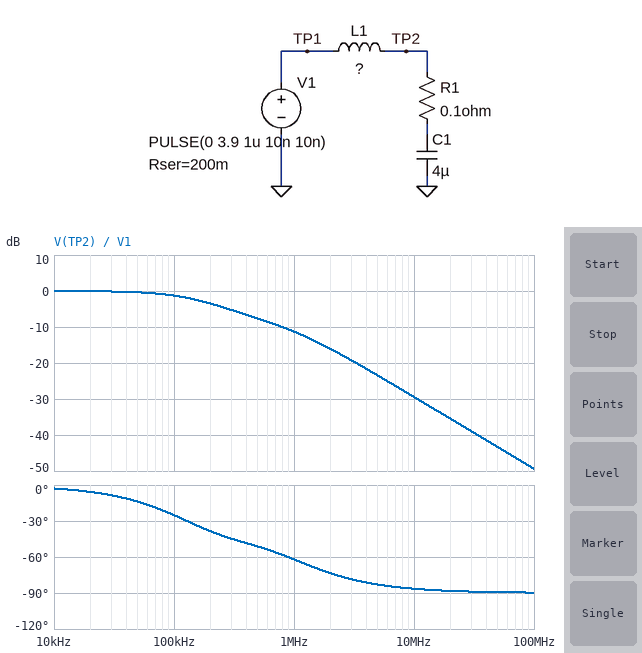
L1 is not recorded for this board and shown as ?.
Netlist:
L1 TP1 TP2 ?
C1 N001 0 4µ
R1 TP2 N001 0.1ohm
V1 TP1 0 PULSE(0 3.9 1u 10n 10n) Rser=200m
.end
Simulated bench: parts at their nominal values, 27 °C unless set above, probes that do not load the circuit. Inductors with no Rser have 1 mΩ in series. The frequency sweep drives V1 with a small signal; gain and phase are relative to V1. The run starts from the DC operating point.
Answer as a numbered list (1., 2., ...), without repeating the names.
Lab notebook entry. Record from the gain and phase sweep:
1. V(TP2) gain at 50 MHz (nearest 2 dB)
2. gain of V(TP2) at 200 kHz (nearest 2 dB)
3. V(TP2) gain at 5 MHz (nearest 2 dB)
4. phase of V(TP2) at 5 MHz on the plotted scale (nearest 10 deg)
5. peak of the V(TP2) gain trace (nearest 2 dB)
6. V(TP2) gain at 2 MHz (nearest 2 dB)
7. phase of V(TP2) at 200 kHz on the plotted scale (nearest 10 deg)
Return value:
1. -44 dB
2. -4 dB
3. -24 dB
4. -80 deg
5. 0 dB
6. -16 dB
7. -40 deg
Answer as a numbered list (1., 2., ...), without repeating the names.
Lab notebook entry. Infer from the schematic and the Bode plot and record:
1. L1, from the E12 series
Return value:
1. 47 nH
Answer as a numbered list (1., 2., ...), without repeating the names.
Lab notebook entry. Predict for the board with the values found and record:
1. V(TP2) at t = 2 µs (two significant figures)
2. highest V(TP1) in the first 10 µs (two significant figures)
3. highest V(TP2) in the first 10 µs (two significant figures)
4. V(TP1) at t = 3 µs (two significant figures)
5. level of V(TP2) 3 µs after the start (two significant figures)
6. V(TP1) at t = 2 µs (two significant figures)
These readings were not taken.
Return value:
1. 2.8 V
2. 3.9 V
3. 3.9 V
4. 3.4 V
5. 3.5 V
6. 2.5 V
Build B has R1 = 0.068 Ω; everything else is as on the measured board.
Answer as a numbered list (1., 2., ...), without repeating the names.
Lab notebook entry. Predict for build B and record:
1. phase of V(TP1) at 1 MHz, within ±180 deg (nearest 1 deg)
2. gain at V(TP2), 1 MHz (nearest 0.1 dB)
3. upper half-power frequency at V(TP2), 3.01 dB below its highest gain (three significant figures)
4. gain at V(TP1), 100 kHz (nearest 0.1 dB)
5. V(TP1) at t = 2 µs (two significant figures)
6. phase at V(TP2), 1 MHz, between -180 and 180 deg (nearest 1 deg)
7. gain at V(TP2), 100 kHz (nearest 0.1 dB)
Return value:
1. 31 deg
2. -13.5 dB
3. 192 kHz
4. -1.7 dB
5. 2.4 V
6. -74 deg
7. -1.1 dB
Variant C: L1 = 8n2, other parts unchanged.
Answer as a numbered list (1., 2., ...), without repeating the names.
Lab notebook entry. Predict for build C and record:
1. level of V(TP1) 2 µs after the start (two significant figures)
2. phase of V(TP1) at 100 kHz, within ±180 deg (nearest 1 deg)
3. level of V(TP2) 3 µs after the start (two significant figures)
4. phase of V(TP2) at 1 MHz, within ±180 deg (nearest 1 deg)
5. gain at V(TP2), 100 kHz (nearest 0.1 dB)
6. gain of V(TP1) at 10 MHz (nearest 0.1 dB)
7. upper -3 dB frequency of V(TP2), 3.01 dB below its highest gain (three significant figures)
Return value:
1. 2.7 V
2. -23 deg
3. 3.4 V
4. -24 deg
5. -1.6 dB
6. -1.1 dB
7. 154 kHz
